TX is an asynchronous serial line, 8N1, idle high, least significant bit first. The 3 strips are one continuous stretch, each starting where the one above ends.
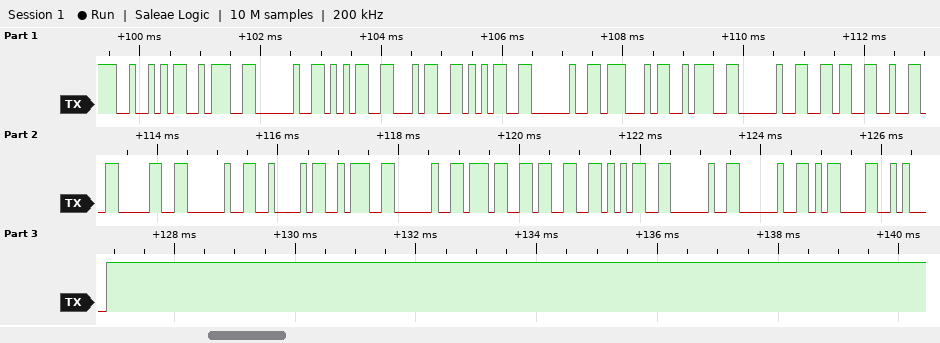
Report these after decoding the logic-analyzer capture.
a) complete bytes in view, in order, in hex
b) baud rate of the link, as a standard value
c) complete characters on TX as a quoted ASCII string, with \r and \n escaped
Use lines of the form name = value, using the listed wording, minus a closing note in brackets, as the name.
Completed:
complete bytes in view, in order, in hex = 52 3A 20 35 34 35 20 47 3A 20 36 32 30 20 42 3A 20 37 33 35 20 20 0D 0A
baud rate of the link, as a standard value = 9600 baud
complete characters on TX as a quoted ASCII string, with \r and \n escaped = "R: 545 G: 620 B: 735  \r\n"
